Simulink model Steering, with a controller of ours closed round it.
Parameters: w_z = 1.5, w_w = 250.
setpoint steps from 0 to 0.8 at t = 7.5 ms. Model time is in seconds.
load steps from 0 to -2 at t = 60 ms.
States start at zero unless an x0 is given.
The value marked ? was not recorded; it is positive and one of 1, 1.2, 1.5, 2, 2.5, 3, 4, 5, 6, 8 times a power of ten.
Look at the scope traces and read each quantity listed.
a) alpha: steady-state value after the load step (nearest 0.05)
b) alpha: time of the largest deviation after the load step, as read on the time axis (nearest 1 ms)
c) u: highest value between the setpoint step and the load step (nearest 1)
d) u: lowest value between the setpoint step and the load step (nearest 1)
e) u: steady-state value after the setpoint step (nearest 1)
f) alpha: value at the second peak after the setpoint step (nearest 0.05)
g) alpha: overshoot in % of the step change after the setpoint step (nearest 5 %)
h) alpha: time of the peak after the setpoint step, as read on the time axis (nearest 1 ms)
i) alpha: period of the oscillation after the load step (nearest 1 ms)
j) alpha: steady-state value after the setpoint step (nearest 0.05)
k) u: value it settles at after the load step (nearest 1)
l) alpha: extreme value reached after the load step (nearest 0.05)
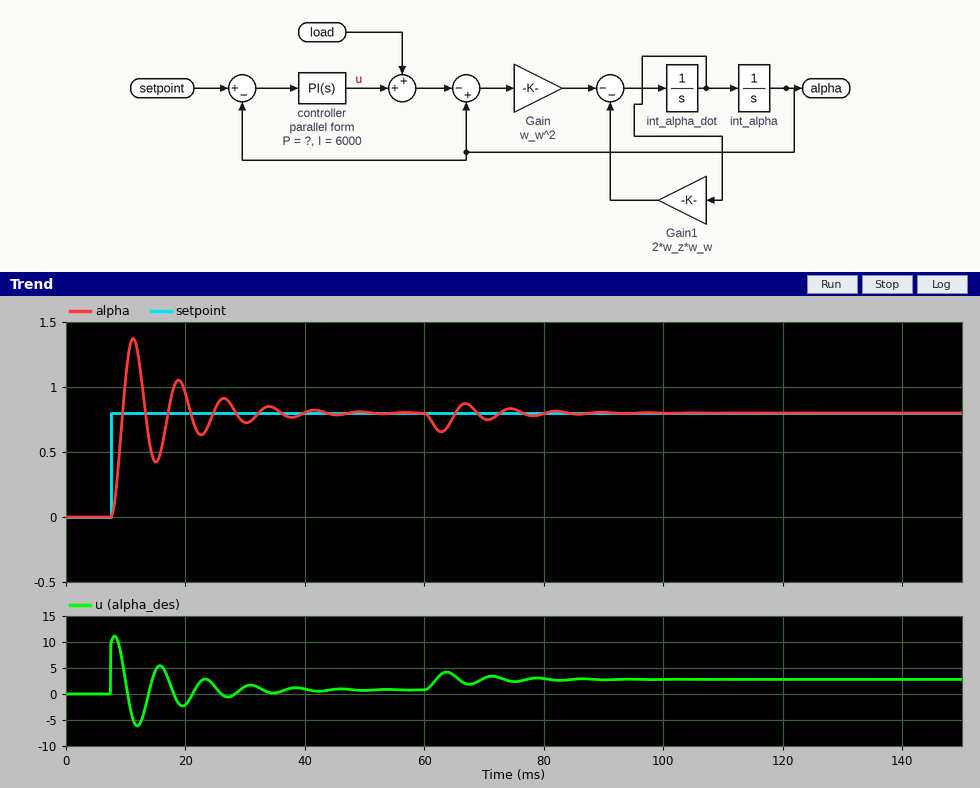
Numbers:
0.80
63 ms
11
-6
1
1.05
70 %
11 ms
8 ms
0.80
3
0.65
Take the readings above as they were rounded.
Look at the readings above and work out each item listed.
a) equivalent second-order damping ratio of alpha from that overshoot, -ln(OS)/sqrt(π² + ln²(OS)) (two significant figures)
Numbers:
0.11
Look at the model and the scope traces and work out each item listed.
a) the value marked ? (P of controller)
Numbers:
12
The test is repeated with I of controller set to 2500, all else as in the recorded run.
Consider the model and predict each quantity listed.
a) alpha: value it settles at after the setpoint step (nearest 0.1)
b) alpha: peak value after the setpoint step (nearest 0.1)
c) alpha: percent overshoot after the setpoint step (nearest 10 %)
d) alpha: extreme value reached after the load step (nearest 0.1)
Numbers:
0.8
1.1
40 %
0.6
